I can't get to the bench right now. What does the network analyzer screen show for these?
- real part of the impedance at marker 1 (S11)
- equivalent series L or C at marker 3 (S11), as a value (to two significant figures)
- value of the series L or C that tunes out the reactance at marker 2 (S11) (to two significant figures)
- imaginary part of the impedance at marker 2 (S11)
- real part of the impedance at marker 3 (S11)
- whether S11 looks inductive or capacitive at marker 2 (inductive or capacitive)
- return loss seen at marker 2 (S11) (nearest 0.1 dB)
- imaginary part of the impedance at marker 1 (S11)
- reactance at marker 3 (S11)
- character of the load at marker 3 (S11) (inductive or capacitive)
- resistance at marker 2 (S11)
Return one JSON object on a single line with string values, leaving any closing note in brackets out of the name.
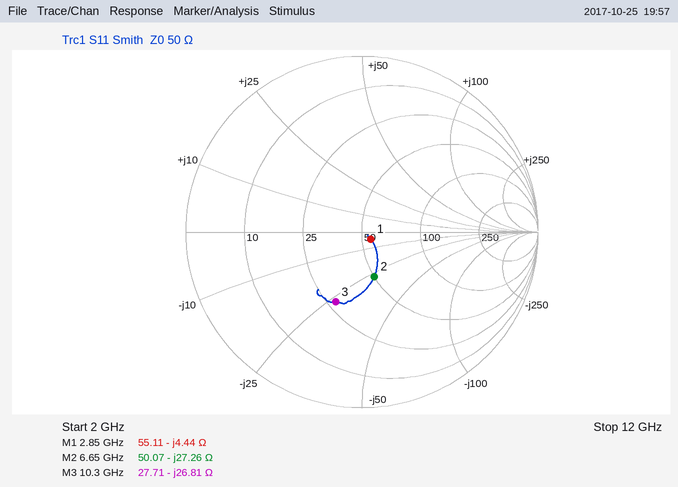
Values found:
{"real part of the impedance at marker 1": "55.11 Ω", "equivalent series L or C at marker 3 (S11), as a value": "580 fF", "value of the series L or C that tunes out the reactance at marker 2 (S11)": "650 pH", "imaginary part of the impedance at marker 2": "-27.26 Ω", "real part of the impedance at marker 3": "27.71 Ω", "whether S11 looks inductive or capacitive at marker 2": "capacitive", "return loss seen at marker 2 (S11)": "11.6 dB", "imaginary part of the impedance at marker 1": "-4.44 Ω", "reactance at marker 3": "-26.81 Ω", "character of the load at marker 3 (S11)": "capacitive", "resistance at marker 2": "50.07 Ω"}
